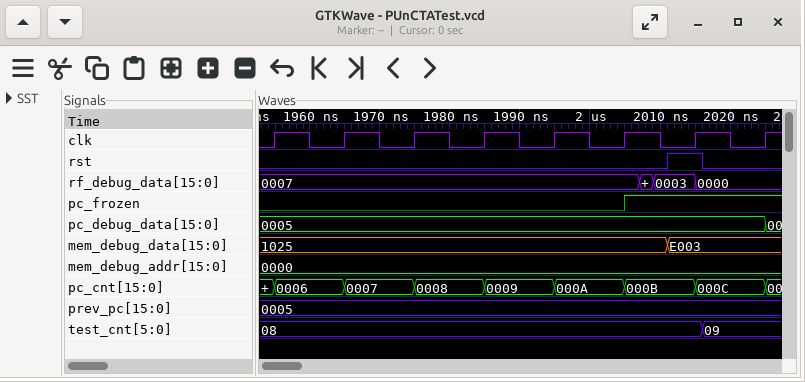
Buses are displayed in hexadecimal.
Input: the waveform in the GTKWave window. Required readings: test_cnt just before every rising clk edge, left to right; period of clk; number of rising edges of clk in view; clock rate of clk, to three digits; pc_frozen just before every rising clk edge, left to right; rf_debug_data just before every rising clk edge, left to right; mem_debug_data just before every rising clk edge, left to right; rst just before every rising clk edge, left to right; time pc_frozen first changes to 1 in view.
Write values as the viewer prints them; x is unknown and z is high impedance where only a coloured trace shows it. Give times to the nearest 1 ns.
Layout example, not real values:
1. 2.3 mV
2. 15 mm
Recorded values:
1. 08, 08, 08, 08, 08, 08, 08, 09
2. 10 ns
3. 8
4. 100 MHz
5. 0 0 0 0 0 0 1 1
6. 0007, 0007, 0007, 0007, 0007, 0007, 0003, 0000
7. 1025, 1025, 1025, 1025, 1025, 1025, E003, E003
8. 0 0 0 0 0 0 1 0
9. 2005 ns
